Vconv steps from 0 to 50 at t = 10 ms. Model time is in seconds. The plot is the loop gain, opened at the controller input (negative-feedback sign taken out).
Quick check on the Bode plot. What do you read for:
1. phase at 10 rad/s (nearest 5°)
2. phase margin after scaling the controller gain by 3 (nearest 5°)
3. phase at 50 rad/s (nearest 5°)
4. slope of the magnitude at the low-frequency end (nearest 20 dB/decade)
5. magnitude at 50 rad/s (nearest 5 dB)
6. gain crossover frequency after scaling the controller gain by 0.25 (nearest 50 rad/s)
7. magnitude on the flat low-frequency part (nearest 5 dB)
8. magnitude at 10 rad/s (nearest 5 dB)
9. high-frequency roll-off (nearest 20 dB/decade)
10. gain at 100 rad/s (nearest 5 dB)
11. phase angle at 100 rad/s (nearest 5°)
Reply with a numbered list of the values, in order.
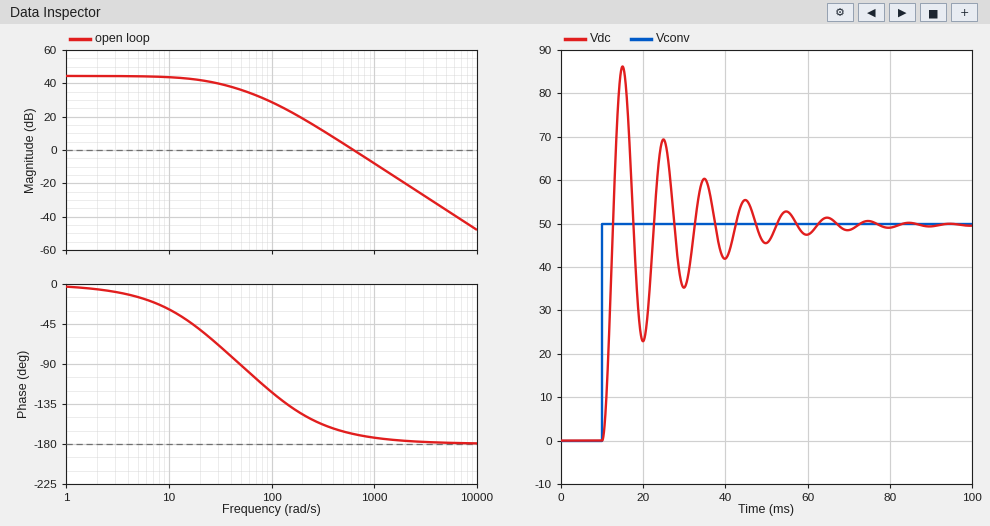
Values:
1. -30°
2. 5°
3. -90°
4. 0 dB/decade
5. 35 dB
6. 300 rad/s
7. 45 dB
8. 45 dB
9. -40 dB/decade
10. 30 dB
11. -120°
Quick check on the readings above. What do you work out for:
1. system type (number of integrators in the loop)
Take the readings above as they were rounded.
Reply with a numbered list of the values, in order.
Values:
1. 0
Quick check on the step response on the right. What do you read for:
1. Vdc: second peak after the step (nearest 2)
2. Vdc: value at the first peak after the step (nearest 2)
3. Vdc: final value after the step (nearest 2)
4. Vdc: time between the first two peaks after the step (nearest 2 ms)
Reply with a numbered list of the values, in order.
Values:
1. 70
2. 86
3. 50
4. 10 ms
